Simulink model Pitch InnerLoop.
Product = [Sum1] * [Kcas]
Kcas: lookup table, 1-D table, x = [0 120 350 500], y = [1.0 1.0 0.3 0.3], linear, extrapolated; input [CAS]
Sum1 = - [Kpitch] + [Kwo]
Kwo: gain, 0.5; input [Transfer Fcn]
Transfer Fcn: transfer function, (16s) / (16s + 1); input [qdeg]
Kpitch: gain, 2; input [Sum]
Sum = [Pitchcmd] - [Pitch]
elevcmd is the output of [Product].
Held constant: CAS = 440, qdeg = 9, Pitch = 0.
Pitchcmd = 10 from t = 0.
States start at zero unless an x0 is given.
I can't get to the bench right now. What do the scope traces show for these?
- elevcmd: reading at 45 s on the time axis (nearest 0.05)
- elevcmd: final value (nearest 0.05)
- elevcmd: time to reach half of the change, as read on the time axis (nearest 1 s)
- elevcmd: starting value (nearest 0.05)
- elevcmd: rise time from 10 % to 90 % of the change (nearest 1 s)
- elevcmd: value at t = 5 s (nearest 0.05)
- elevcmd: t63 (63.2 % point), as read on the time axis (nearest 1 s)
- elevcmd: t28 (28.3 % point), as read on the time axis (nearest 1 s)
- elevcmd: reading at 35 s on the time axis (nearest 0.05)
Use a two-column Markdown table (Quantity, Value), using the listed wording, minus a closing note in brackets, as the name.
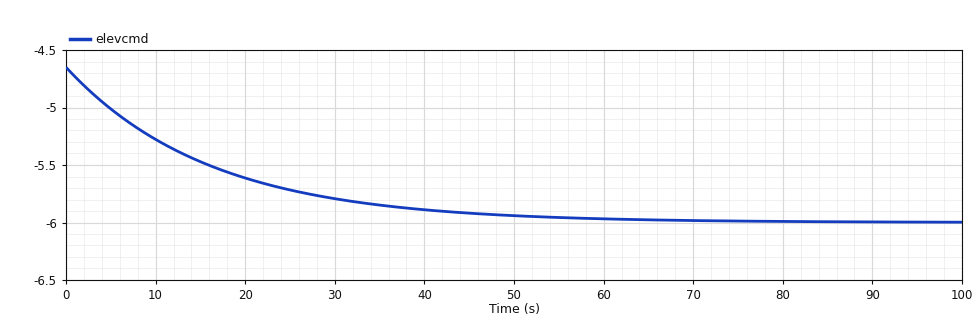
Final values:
| Quantity | Value |
|---|---|
| elevcmd: reading at 45 s on the time axis | -5.90 |
| elevcmd: final value | -6.00 |
| elevcmd: time to reach half of the change, as read on the time axis | 11 s |
| elevcmd: starting value | -4.65 |
| elevcmd: rise time from 10 % to 90 % of the change | 35 s |
| elevcmd: value at t = 5 s | -5.00 |
| elevcmd: t63 (63.2 % point), as read on the time axis | 16 s |
| elevcmd: t28 (28.3 % point), as read on the time axis | 5 s |
| elevcmd: reading at 35 s on the time axis | -5.85 |
